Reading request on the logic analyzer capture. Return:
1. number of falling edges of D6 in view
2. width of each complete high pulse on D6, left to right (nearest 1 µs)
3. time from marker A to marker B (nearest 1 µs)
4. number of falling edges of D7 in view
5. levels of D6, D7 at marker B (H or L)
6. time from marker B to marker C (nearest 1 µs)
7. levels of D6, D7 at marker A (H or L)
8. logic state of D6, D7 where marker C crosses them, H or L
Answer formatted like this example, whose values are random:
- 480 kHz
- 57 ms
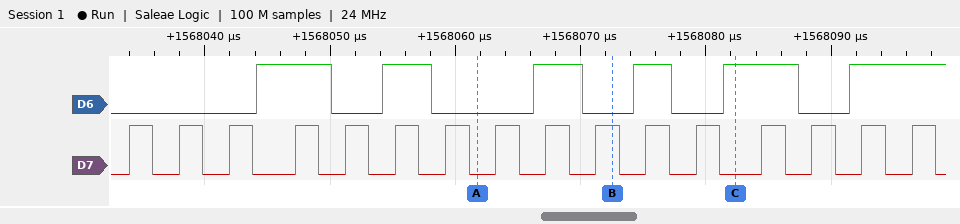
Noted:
- 5
- 6 µs, 4 µs, 4 µs, 3 µs, 6 µs
- 11 µs
- 16
- D6=L, D7=H
- 10 µs
- D6=L, D7=L
- D6=H, D7=L
